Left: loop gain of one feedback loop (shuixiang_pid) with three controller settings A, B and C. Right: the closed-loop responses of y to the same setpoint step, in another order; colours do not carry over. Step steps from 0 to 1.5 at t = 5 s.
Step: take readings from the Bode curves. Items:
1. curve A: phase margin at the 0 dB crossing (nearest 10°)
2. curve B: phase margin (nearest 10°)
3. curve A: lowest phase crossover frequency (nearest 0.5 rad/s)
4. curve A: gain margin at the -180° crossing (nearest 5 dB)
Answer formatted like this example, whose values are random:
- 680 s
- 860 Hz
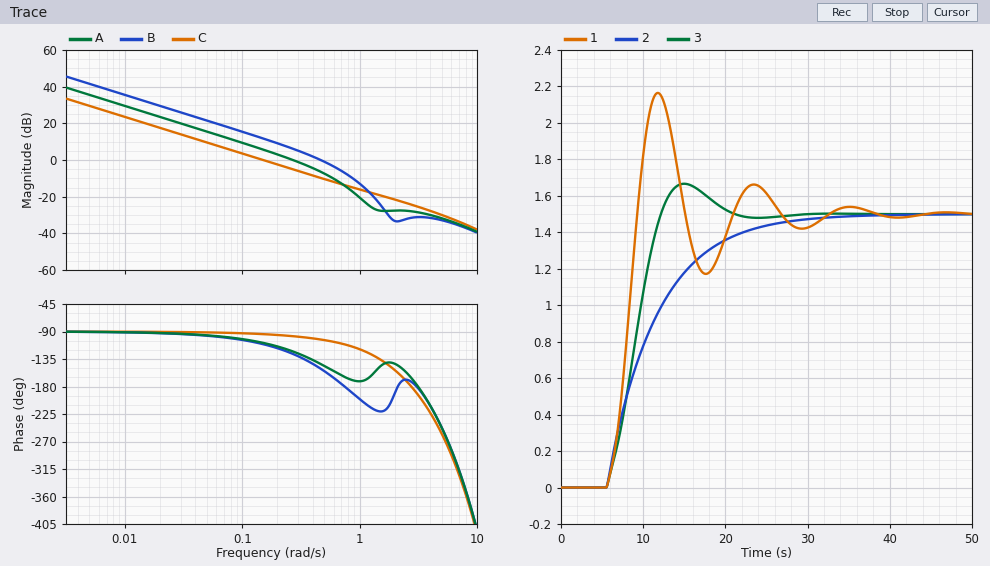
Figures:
- 60°
- 30°
- 3.0 rad/s
- 30 dB
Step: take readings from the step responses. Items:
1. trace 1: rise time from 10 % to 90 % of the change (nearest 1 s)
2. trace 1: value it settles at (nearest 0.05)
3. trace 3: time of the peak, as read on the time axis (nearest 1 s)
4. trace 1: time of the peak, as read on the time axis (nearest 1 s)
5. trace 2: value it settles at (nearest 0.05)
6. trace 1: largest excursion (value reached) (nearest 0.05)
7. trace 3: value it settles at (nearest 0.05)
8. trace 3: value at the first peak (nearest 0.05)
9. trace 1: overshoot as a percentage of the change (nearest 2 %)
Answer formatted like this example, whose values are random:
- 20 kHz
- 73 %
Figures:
- 3 s
- 1.50
- 15 s
- 12 s
- 1.50
- 2.15
- 1.50
- 1.65
- 44 %
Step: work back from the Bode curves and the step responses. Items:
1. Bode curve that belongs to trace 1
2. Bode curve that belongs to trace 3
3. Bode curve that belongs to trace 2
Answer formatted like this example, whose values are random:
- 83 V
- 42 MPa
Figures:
- B
- A
- C
